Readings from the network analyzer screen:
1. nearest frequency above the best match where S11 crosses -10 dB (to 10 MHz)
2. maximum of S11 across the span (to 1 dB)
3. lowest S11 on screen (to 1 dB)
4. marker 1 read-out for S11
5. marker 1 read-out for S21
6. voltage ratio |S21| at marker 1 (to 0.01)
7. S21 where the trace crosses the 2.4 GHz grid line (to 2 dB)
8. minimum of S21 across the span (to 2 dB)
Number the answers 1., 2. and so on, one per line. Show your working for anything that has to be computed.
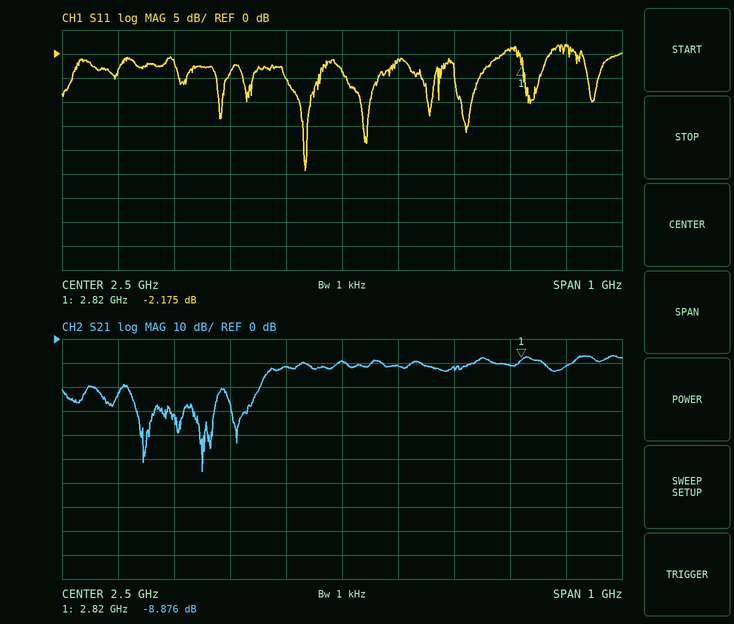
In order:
1. 2.44 GHz
2. 2 dB
3. -24 dB
4. -2.175 dB
5. -8.876 dB
6. 10^(-8.876/20) ≈ 0.36
7. -12 dB
8. -56 dB
